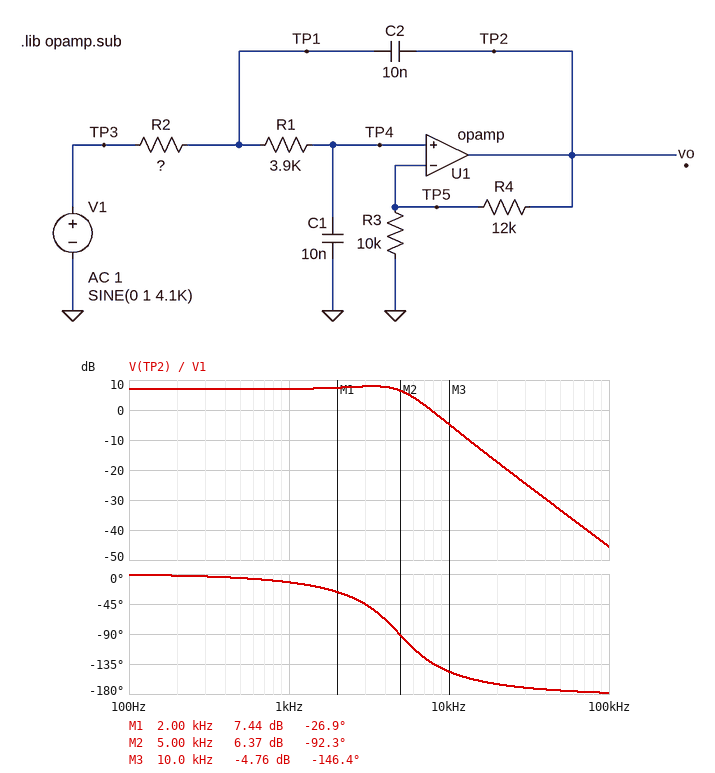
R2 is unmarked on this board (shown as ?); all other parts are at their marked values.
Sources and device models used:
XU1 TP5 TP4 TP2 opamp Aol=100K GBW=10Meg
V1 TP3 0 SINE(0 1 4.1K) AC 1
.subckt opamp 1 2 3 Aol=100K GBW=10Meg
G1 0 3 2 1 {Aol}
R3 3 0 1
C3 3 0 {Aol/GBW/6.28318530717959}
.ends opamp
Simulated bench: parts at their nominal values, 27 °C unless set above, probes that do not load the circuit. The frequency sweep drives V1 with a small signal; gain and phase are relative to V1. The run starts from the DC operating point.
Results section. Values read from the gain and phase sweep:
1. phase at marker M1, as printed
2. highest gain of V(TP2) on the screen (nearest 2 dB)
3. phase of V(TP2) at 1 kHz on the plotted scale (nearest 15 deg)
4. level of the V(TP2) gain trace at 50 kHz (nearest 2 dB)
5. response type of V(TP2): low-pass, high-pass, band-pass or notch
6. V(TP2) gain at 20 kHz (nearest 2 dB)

-26.9 deg
8 dB
-15 deg
-34 dB
low-pass
-18 dB
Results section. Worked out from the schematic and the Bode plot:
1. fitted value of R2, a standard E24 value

2.7 kΩ
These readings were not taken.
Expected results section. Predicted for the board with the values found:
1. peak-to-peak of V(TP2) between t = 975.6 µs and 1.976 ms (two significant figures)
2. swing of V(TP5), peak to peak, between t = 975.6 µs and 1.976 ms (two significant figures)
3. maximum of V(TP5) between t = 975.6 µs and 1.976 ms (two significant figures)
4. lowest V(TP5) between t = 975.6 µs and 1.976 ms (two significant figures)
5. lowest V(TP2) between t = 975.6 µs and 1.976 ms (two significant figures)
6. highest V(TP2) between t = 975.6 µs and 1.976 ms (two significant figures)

4.8 V
2.2 V
1.1 V
-1.1 V
-2.4 V
2.4 V
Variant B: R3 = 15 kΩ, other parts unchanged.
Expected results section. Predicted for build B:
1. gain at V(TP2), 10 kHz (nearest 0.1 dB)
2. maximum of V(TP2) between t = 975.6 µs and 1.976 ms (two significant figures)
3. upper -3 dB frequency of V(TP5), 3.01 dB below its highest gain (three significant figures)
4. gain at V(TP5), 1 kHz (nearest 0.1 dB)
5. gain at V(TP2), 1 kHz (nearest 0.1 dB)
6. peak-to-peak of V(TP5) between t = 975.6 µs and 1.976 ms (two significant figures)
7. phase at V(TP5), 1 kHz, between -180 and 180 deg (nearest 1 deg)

-7.4 dB
1.5 V
5.05 kHz
0 dB
5.1 dB
1.7 V
-16 deg
